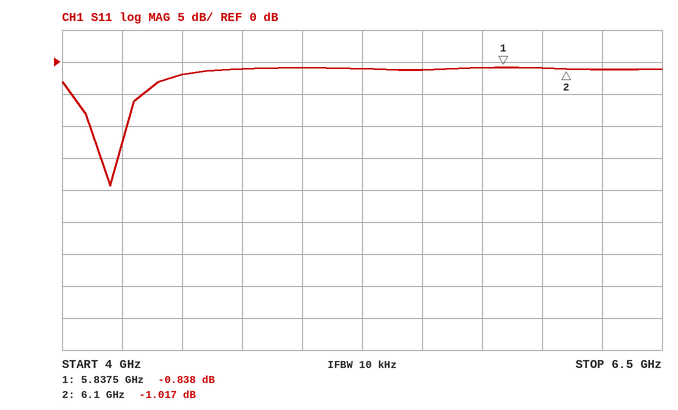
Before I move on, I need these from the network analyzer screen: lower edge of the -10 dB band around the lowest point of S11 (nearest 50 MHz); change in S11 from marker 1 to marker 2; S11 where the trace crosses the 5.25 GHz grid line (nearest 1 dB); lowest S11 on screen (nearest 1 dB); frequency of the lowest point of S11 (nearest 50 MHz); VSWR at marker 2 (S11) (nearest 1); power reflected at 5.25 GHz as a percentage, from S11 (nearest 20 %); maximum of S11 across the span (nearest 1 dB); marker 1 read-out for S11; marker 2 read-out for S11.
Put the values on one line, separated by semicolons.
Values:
4.10 GHz; -0.179 dB; -1 dB; -19 dB; 4.20 GHz; 17; 80 %; -1 dB; -0.838 dB; -1.017 dB
